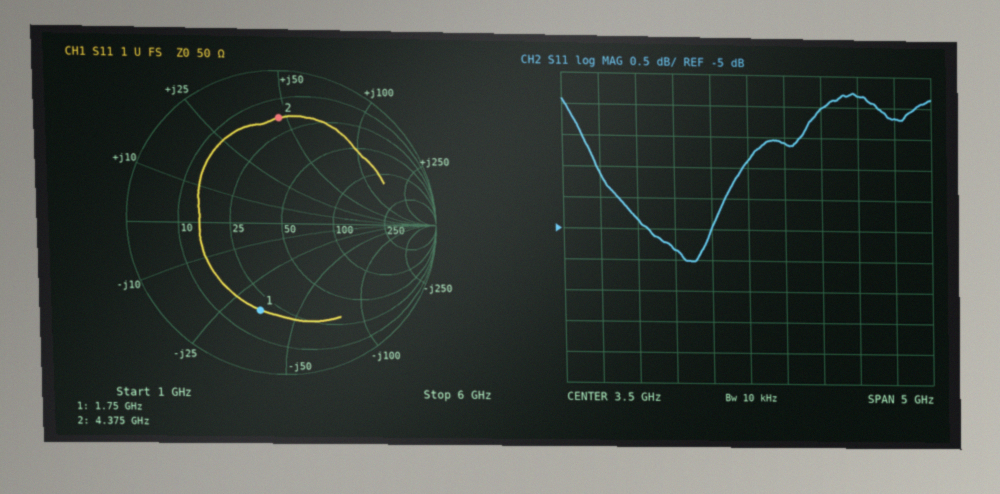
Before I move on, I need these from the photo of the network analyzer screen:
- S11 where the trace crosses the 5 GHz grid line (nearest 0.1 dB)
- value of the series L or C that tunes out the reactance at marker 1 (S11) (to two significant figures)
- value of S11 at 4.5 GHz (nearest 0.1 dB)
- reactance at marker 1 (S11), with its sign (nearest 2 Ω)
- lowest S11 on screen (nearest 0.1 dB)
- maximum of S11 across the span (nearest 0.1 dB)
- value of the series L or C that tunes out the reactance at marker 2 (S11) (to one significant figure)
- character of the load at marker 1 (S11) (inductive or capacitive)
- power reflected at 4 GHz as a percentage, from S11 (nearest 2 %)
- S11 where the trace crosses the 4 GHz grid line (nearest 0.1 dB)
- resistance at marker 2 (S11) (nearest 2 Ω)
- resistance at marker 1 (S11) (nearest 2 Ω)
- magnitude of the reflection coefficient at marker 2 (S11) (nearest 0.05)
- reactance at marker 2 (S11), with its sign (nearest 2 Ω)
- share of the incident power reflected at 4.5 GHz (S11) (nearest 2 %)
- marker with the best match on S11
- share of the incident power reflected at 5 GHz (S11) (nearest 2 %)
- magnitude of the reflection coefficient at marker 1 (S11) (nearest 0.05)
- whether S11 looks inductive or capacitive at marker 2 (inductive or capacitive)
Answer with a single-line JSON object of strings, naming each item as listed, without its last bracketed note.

{"S11 where the trace crosses the 5 GHz grid line": "-2.8 dB", "value of the series L or C that tunes out the reactance at marker 1 (S11)": "3.1 nH", "value of S11 at 4.5 GHz": "-3.0 dB", "reactance at marker 1 (S11), with its sign": "-34 Ω", "lowest S11 on screen": "-5.5 dB", "maximum of S11 across the span": "-2.8 dB", "value of the series L or C that tunes out the reactance at marker 2 (S11)": "800 fF", "character of the load at marker 1 (S11)": "capacitive", "power reflected at 4 GHz as a percentage, from S11": "44 %", "S11 where the trace crosses the 4 GHz grid line": "-3.6 dB", "resistance at marker 2 (S11)": "18 Ω", "resistance at marker 1 (S11)": "20 Ω", "magnitude of the reflection coefficient at marker 2 (S11)": "0.70", "reactance at marker 2 (S11), with its sign": "+46 Ω", "share of the incident power reflected at 4.5 GHz (S11)": "50 %", "marker with the best match on S11": "marker 1", "share of the incident power reflected at 5 GHz (S11)": "52 %", "magnitude of the reflection coefficient at marker 1 (S11)": "0.60", "whether S11 looks inductive or capacitive at marker 2": "inductive"}
